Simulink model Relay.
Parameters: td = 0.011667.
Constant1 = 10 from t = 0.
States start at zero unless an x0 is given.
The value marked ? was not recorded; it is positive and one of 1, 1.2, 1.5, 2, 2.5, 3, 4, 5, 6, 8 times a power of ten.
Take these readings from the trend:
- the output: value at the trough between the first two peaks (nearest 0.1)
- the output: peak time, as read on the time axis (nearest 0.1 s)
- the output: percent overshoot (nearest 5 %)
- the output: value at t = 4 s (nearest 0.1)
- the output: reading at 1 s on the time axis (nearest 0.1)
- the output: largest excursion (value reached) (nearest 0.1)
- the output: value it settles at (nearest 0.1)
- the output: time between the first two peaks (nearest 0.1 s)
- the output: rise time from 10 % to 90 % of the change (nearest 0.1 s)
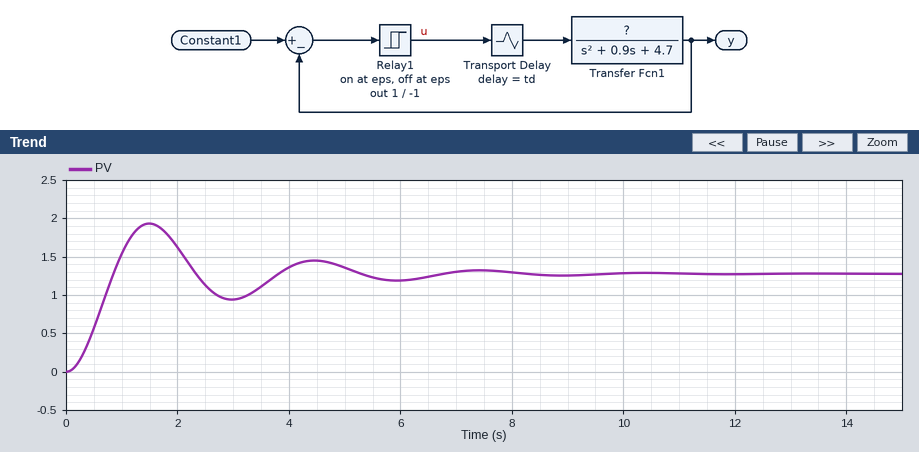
0.9
1.5 s
50 %
1.4
1.5
1.9
1.3
3.0 s
0.6 s
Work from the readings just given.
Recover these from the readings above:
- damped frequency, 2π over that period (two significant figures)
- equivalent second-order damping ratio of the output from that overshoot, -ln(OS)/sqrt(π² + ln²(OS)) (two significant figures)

2.1 rad/s
0.22
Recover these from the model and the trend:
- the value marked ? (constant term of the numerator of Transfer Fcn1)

6
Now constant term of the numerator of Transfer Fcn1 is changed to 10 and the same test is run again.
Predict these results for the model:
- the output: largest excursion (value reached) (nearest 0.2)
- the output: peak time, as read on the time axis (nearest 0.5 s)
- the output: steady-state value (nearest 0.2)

3.2
1.5 s
2.2
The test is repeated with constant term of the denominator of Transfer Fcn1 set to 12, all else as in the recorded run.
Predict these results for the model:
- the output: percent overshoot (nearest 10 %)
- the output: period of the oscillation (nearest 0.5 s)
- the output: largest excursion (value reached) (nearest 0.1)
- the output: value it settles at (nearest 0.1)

70 %
2.0 s
0.8
0.5
